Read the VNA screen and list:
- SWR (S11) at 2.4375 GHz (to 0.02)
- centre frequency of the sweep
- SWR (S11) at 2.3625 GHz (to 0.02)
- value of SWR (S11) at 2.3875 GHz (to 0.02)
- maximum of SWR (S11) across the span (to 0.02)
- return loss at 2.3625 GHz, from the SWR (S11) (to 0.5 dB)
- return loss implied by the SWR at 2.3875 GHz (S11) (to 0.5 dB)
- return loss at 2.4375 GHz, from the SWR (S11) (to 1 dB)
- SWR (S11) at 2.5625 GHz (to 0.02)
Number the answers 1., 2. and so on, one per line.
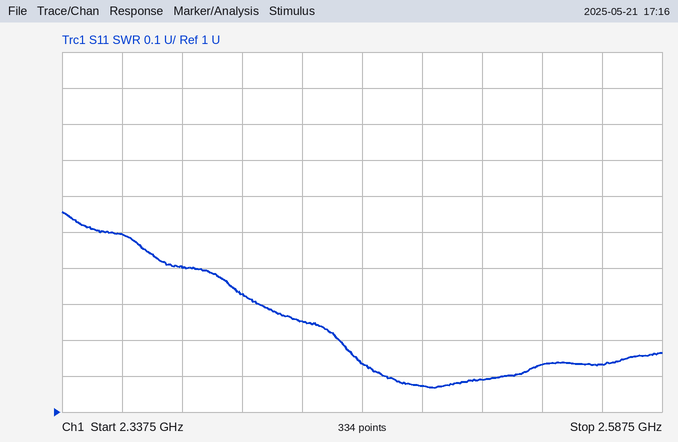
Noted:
1. 1.26
2. 2.4625 GHz
3. 1.50
4. 1.40
5. 1.56
6. 14.0 dB
7. 15.5 dB
8. 19 dB
9. 1.14
